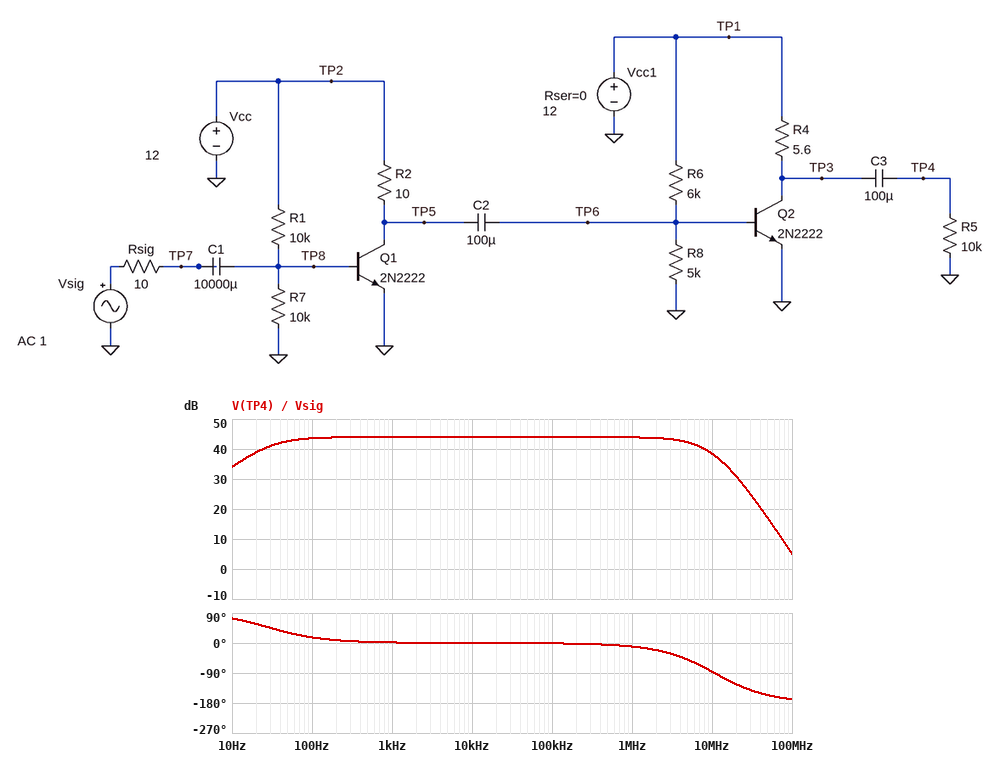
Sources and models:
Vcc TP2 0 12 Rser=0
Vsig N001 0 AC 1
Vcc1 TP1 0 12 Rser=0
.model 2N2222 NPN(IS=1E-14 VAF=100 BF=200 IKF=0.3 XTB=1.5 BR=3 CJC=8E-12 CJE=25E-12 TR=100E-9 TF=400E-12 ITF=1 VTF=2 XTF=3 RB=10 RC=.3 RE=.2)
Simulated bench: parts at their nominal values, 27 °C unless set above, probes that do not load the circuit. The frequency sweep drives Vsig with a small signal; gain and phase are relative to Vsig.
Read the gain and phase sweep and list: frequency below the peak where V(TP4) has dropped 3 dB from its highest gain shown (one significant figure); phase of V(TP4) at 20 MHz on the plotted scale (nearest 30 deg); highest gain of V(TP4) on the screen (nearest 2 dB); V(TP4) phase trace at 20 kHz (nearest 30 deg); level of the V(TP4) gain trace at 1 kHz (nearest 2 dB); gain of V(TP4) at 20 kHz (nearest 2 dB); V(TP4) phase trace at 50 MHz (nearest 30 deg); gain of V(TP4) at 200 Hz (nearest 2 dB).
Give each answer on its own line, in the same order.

30 Hz
-120 deg
44 dB
0 deg
44 dB
44 dB
-150 deg
44 dB
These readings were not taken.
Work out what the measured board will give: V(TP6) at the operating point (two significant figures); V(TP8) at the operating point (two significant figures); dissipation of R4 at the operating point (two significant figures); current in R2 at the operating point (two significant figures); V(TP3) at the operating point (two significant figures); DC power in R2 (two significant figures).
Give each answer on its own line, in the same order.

870 mV
830 mV
270 mW
150 mA
11 V
240 mW
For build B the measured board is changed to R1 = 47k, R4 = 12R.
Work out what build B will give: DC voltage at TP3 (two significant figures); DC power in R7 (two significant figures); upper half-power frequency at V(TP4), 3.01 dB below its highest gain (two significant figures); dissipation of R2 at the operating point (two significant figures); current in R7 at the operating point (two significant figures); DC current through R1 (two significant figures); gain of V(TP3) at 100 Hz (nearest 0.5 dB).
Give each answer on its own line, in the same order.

9.4 V
57 µW
8.3 MHz
11 mW
75 µA
240 µA
44.5 dB
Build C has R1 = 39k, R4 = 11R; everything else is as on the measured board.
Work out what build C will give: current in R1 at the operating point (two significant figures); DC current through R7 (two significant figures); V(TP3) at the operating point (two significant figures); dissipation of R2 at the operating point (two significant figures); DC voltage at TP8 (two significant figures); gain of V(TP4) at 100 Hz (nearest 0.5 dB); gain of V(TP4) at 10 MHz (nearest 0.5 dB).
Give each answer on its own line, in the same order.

290 µA
76 µA
9.6 V
17 mW
760 mV
45.0 dB
41.0 dB
